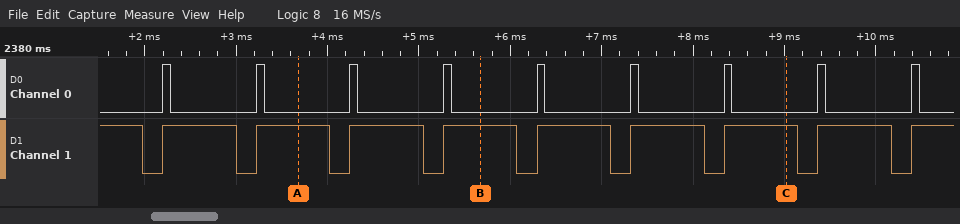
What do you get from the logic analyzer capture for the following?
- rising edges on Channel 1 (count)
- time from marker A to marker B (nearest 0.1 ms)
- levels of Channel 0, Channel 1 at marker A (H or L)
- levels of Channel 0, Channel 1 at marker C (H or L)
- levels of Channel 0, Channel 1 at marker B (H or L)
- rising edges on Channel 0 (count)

9
2 ms
Channel 0=L, Channel 1=H
Channel 0=L, Channel 1=H
Channel 0=L, Channel 1=H
9
